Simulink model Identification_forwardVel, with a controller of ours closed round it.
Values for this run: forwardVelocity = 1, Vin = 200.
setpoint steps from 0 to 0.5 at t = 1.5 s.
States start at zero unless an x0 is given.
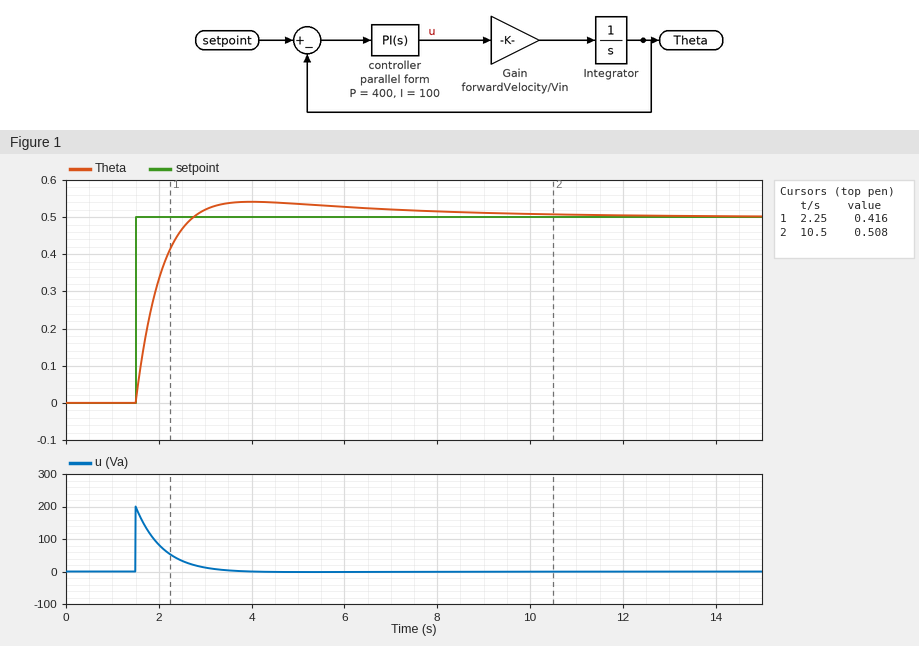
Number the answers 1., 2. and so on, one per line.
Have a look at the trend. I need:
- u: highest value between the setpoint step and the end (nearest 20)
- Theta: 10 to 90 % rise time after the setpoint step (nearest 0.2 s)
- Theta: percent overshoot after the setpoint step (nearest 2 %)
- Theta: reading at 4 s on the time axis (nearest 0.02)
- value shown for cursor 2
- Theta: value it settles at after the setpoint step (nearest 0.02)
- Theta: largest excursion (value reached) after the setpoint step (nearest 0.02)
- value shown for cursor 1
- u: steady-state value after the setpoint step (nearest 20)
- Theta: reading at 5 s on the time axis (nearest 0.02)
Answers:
1. 200
2. 0.8 s
3. 8 %
4. 0.54
5. 0.508
6. 0.50
7. 0.54
8. 0.416
9. 0
10. 0.54
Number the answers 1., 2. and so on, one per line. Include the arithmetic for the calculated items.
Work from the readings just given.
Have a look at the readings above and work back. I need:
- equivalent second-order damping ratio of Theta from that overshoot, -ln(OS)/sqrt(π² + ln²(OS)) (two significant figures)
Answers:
1. ln(0.08) = -2.526; 2.526 / sqrt(9.870 + 6.379) = 0.63
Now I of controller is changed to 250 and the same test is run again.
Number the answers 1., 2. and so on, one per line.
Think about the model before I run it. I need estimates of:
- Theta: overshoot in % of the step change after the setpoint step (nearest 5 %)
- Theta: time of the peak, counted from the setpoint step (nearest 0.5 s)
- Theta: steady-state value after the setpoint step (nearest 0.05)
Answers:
1. 15 %
2. 2.0 s
3. 0.50
